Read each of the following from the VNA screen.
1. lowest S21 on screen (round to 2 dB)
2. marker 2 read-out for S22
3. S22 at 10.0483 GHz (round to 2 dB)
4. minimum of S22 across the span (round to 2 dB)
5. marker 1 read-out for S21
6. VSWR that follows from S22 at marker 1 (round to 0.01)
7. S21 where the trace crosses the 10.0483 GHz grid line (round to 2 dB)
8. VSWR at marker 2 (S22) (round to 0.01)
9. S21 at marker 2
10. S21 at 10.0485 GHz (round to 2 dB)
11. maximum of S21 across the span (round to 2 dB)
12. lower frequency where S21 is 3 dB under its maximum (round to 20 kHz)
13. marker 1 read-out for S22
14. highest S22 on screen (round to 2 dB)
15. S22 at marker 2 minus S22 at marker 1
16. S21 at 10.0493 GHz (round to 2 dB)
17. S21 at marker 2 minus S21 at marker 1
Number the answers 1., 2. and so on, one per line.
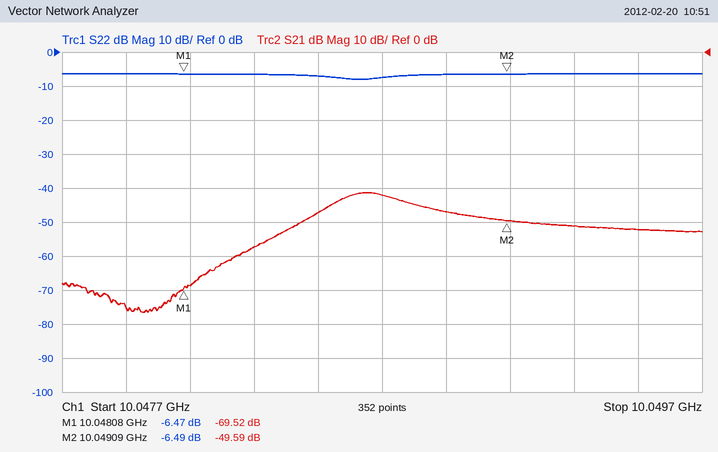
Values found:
1. -76 dB
2. -6.49 dB
3. -6 dB
4. -8 dB
5. -69.52 dB
6. 2.81
7. -58 dB
8. 2.80
9. -49.59 dB
10. -48 dB
11. -42 dB
12. 10.04856 GHz
13. -6.47 dB
14. -6 dB
15. -0.02 dB
16. -52 dB
17. 19.93 dB
